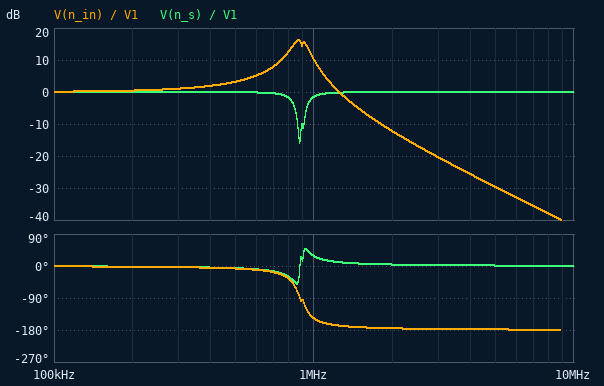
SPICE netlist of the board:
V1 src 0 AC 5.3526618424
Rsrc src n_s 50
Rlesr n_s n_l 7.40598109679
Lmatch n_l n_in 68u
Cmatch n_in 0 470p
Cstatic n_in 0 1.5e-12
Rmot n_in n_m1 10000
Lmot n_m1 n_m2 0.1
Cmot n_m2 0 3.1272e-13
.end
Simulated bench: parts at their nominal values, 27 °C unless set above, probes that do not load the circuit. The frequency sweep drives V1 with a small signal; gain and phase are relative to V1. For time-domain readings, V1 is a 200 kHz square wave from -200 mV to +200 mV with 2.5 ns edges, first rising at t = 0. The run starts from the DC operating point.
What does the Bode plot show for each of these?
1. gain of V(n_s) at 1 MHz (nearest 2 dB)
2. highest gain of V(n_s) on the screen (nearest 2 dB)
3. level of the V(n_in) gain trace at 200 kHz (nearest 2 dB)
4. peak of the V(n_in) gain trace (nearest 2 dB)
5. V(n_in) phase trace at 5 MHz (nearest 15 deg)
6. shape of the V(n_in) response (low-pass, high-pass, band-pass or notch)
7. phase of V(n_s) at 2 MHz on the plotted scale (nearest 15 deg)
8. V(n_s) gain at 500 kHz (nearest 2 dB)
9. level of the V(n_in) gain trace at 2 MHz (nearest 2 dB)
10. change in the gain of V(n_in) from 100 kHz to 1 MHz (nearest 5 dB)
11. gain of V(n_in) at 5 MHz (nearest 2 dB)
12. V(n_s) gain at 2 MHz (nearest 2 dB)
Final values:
-2 dB
0 dB
0 dB
16 dB
-180 deg
low-pass
0 deg
0 dB
-12 dB
10 dB
-30 dB
0 dB
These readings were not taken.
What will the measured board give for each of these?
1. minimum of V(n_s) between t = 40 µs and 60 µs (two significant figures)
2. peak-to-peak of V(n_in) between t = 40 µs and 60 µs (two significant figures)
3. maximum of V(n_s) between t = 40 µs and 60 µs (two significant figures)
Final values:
-230 mV
950 mV
230 mV
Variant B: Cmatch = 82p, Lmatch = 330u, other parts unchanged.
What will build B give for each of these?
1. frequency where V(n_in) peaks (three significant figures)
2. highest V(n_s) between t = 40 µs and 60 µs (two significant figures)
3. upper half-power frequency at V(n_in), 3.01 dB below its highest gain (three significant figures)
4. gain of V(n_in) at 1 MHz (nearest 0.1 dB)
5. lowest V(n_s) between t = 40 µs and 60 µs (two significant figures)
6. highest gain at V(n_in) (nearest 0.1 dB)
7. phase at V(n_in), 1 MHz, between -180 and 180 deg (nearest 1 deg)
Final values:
970 kHz
220 mV
983 kHz
22.3 dB
-220 mV
30.1 dB
-156 deg
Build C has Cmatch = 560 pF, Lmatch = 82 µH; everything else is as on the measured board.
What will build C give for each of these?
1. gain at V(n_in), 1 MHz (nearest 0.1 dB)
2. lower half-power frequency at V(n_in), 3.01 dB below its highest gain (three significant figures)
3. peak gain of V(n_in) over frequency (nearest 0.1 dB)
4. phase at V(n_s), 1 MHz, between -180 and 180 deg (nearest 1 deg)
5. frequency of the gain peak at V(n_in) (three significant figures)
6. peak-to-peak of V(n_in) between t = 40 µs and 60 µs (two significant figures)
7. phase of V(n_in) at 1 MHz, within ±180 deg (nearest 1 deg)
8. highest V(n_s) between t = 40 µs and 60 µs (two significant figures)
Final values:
1.5 dB
679 kHz
16.5 dB
12 deg
737 kHz
900 mV
-166 deg
230 mV
